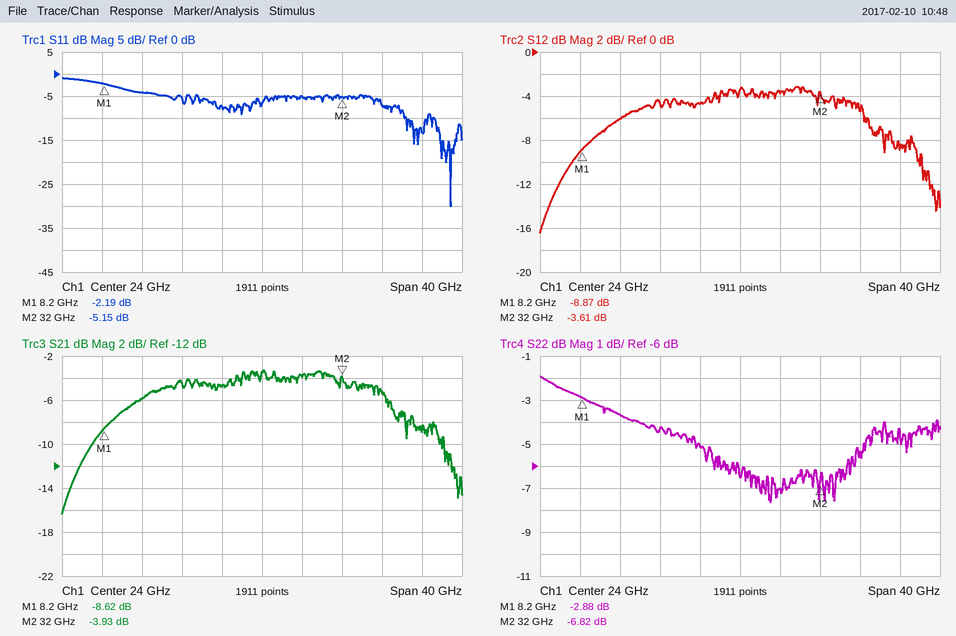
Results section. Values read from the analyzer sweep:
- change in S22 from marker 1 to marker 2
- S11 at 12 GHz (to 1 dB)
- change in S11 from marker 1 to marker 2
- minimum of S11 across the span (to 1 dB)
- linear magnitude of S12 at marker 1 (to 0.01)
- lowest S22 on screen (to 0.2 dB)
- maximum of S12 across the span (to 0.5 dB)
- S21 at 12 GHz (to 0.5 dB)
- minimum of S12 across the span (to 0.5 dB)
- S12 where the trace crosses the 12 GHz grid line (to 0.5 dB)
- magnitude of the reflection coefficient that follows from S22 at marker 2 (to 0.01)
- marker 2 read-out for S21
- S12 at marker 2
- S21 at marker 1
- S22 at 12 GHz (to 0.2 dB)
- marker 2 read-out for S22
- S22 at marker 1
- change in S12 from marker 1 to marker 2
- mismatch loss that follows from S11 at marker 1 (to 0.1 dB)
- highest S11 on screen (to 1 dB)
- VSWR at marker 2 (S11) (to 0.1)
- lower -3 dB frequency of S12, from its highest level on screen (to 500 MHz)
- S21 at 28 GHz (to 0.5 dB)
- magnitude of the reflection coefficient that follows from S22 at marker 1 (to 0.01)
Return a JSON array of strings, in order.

["-3.94 dB", "-4 dB", "-2.96 dB", "-30 dB", "0.36", "-7.6 dB", "-3.0 dB", "-6.0 dB", "-16.5 dB", "-6.0 dB", "0.46", "-3.93 dB", "-3.61 dB", "-8.62 dB", "-3.6 dB", "-6.82 dB", "-2.88 dB", "5.26 dB", "4.0 dB", "-1 dB", "3.5", "12.0 GHz", "-4.0 dB", "0.72"]
